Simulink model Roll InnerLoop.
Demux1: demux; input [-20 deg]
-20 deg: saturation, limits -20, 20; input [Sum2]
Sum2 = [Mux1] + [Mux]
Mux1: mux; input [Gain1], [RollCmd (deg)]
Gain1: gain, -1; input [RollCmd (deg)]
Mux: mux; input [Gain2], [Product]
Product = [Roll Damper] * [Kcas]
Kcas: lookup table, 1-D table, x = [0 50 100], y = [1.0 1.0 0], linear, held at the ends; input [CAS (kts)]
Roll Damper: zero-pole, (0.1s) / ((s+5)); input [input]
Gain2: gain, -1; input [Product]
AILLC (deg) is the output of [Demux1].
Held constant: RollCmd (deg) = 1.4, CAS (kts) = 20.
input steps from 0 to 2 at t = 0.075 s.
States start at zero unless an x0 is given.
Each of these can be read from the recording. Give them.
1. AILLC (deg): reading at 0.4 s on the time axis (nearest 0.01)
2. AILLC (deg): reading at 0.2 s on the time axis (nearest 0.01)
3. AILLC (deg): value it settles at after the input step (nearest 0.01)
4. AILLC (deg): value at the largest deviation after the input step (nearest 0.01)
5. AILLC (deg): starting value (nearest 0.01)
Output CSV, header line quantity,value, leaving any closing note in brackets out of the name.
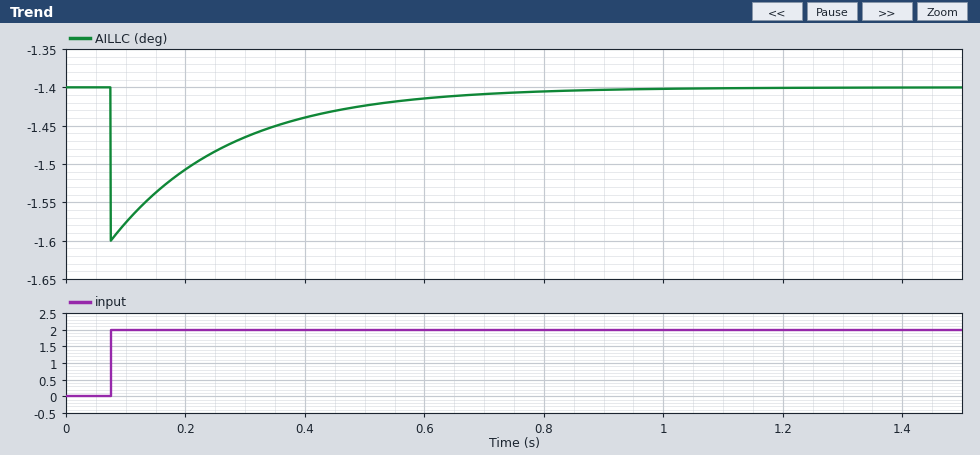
quantity,value
AILLC (deg): reading at 0.4 s on the time axis,-1.44
AILLC (deg): reading at 0.2 s on the time axis,-1.51
AILLC (deg): value it settles at after the input step,-1.40
AILLC (deg): value at the largest deviation after the input step,-1.60
AILLC (deg): starting value,-1.40
